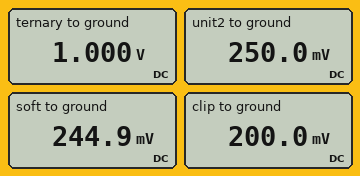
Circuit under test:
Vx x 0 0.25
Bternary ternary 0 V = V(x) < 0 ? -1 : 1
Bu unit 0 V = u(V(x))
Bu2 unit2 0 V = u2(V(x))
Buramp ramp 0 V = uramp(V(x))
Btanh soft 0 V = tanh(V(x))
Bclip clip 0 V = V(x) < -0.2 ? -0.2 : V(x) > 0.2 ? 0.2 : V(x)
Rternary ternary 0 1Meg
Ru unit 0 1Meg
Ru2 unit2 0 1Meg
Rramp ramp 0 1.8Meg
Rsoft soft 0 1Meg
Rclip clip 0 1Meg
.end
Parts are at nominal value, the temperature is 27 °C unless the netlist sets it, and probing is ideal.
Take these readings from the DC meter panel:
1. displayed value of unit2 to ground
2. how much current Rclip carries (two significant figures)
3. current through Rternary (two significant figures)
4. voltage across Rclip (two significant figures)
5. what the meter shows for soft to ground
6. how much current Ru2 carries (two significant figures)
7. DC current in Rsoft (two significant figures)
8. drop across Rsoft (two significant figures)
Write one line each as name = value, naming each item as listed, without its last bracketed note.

displayed value of unit2 to ground = 250.0 mV
how much current Rclip carries = 200 nA
current through Rternary = 1.0 µA
voltage across Rclip = 200 mV
what the meter shows for soft to ground = 244.9 mV
how much current Ru2 carries = 250 nA
DC current in Rsoft = 240 nA
drop across Rsoft = 240 mV
